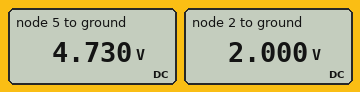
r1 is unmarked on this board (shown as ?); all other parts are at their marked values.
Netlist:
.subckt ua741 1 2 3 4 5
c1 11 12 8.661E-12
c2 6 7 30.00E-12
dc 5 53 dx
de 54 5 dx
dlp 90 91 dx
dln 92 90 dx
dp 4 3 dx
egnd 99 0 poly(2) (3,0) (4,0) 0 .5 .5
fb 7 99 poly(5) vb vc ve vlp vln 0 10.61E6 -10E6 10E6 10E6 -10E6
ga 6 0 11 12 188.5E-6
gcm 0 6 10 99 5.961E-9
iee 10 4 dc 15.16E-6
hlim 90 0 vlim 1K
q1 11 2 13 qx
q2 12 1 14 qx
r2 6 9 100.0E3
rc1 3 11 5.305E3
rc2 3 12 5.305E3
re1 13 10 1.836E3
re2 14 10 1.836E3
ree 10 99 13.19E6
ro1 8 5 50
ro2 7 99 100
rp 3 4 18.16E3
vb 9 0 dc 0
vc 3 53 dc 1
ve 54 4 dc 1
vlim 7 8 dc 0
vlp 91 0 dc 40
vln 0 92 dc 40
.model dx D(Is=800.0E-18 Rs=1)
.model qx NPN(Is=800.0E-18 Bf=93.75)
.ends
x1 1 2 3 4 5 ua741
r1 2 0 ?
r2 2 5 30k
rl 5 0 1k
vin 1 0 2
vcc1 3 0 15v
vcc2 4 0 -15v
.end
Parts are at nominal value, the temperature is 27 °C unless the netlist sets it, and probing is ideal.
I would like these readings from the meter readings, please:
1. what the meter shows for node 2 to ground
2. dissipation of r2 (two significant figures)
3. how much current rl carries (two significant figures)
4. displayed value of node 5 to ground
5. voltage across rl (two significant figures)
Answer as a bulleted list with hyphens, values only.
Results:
- 2.000 V
- 250 µW
- 4.7 mA
- 4.730 V
- 4.7 V
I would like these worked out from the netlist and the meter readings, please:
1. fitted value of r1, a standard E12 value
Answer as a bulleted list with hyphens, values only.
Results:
- 22 kΩ
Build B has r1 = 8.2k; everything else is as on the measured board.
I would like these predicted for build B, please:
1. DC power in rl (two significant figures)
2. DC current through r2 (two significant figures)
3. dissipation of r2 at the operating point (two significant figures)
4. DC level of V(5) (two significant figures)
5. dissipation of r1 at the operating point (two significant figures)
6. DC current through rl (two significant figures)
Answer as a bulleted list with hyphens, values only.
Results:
- 87 mW
- 240 µA
- 1.8 mW
- 9.3 V
- 490 µW
- 9.3 mA
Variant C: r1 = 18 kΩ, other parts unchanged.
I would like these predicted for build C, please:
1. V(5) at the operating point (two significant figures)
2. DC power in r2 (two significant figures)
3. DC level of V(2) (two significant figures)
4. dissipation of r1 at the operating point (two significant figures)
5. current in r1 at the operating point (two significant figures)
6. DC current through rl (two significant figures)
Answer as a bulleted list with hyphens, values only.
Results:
- 5.3 V
- 370 µW
- 2.0 V
- 220 µW
- 110 µA
- 5.3 mA
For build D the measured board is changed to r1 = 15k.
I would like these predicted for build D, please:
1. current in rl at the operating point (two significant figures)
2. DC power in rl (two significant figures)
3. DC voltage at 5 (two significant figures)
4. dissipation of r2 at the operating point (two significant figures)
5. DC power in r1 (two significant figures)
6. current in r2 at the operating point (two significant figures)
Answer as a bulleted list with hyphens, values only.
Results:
- 6.0 mA
- 36 mW
- 6.0 V
- 530 µW
- 270 µW
- 130 µA
